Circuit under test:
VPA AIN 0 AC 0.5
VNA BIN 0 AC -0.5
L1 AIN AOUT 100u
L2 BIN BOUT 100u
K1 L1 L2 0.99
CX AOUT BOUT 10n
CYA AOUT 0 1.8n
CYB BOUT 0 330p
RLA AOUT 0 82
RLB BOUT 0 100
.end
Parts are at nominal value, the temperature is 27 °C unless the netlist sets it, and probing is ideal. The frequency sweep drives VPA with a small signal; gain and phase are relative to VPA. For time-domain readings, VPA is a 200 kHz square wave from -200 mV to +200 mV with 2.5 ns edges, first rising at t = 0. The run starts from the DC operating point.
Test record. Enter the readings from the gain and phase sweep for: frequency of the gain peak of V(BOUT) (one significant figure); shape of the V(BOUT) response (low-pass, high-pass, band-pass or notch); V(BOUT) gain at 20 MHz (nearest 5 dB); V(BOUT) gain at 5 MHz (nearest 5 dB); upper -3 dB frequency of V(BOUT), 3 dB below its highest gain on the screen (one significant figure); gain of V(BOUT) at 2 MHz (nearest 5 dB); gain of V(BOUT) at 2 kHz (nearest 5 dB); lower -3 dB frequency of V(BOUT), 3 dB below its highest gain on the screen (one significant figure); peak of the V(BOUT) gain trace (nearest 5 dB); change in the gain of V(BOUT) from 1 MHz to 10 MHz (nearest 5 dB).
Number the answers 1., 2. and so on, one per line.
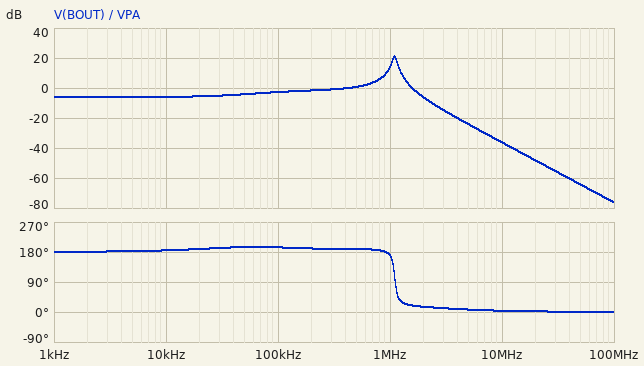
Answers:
1. 1 MHz
2. band-pass
3. -50 dB
4. -25 dB
5. 1 MHz
6. -5 dB
7. -5 dB
8. 1 MHz
9. 20 dB
10. -50 dB
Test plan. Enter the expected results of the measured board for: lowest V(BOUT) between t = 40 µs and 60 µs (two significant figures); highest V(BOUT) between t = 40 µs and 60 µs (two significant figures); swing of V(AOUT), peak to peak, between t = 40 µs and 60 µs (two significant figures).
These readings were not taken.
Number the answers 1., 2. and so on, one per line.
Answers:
1. -360 mV
2. 360 mV
3. 430 mV
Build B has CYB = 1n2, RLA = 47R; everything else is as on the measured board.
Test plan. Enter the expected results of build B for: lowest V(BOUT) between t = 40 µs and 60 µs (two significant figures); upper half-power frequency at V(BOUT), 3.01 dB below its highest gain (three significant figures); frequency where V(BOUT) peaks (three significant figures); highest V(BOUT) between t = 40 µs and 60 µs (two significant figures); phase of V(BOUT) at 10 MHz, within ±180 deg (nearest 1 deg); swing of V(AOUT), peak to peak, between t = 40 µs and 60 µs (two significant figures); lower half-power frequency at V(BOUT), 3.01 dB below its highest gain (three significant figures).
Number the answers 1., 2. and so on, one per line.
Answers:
1. -410 mV
2. 1.13 MHz
3. 1.08 MHz
4. 410 mV
5. -1 deg
6. 350 mV
7. 1.03 MHz
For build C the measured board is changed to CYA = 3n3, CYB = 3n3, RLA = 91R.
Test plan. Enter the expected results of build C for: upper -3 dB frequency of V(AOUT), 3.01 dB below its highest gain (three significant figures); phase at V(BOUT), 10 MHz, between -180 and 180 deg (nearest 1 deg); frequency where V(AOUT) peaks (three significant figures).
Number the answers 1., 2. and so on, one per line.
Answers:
1. 1.08 MHz
2. 0 deg
3. 1.04 MHz
